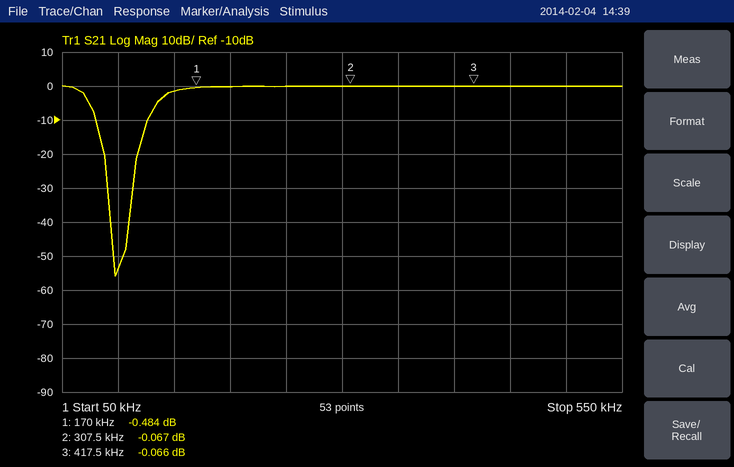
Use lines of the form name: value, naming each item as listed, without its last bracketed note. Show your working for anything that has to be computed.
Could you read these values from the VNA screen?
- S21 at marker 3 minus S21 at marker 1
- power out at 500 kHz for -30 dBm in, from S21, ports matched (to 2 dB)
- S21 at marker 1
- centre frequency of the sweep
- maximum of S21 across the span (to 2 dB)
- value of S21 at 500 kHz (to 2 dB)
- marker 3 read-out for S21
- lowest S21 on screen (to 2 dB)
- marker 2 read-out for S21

S21 at marker 3 minus S21 at marker 1: -0.066 − (-0.484) = 0.418 dB
power out at 500 kHz for -30 dBm in, from S21, ports matched: -30 dBm + (0 dB) = -30 dBm
S21 at marker 1: -0.484 dB
centre frequency of the sweep: 300 kHz
maximum of S21 across the span: 0 dB
value of S21 at 500 kHz: 0 dB
marker 3 read-out for S21: -0.066 dB
lowest S21 on screen: -56 dB
marker 2 read-out for S21: -0.067 dB
